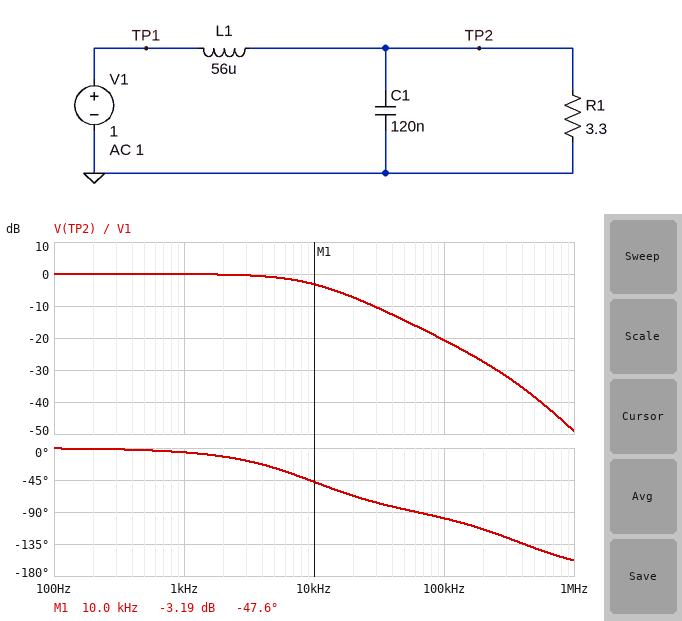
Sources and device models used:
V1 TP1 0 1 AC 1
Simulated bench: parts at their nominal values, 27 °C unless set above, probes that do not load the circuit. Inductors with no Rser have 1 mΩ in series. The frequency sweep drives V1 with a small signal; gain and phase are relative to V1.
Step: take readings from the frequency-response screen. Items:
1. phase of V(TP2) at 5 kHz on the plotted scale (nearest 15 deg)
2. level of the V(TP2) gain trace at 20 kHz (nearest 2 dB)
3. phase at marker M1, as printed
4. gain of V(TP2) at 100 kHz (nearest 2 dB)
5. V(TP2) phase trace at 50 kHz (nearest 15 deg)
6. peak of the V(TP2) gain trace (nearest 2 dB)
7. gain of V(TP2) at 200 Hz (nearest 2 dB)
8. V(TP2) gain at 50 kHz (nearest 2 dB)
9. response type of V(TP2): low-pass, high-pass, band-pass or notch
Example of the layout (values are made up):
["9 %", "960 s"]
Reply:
["-30 deg", "-8 dB", "-47.6 deg", "-20 dB", "-90 deg", "0 dB", "0 dB", "-14 dB", "low-pass"]
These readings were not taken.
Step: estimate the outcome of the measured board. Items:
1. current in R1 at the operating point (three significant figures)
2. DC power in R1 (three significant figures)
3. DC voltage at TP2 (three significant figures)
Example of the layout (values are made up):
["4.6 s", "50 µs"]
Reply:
["303 mA", "303 mW", "1.00 V"]
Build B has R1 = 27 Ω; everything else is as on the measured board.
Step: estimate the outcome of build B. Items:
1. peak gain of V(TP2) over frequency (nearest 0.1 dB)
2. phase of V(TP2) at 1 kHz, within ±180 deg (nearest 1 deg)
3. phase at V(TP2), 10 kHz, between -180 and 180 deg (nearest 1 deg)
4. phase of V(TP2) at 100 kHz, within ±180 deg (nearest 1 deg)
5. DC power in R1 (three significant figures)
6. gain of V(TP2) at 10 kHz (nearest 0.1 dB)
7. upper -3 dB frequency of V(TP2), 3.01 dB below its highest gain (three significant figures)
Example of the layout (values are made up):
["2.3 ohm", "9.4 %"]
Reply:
["2.7 dB", "-1 deg", "-8 deg", "-142 deg", "37.0 mW", "0.2 dB", "73.0 kHz"]
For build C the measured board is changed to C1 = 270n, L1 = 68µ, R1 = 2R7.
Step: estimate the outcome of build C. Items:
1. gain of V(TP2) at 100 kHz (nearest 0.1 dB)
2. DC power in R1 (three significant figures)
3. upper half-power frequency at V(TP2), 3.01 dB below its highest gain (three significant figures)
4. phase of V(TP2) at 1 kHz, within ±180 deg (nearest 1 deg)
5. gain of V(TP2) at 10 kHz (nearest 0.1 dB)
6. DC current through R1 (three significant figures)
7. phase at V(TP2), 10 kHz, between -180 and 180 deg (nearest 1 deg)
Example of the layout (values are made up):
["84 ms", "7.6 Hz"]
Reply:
["-24.6 dB", "370 mW", "6.51 kHz", "-9 deg", "-5.3 dB", "370 mA", "-60 deg"]
